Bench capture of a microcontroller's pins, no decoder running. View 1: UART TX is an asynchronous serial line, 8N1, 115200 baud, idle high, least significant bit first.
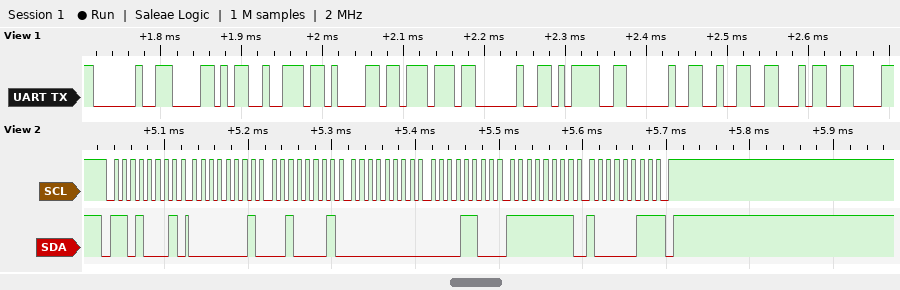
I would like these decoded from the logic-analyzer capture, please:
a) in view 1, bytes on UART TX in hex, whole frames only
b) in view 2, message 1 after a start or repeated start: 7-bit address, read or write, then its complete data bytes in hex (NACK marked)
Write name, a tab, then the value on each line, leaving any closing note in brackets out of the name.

in view 1, bytes on UART TX in hex, whole frames only	20 58 72 61 77 20 3D 20 32 34
in view 2, message 1 after a start or repeated start: 7-bit address, read or write, then its complete data bytes in hex	0x68 read: 01 21 00 0C FF 83 NACK
